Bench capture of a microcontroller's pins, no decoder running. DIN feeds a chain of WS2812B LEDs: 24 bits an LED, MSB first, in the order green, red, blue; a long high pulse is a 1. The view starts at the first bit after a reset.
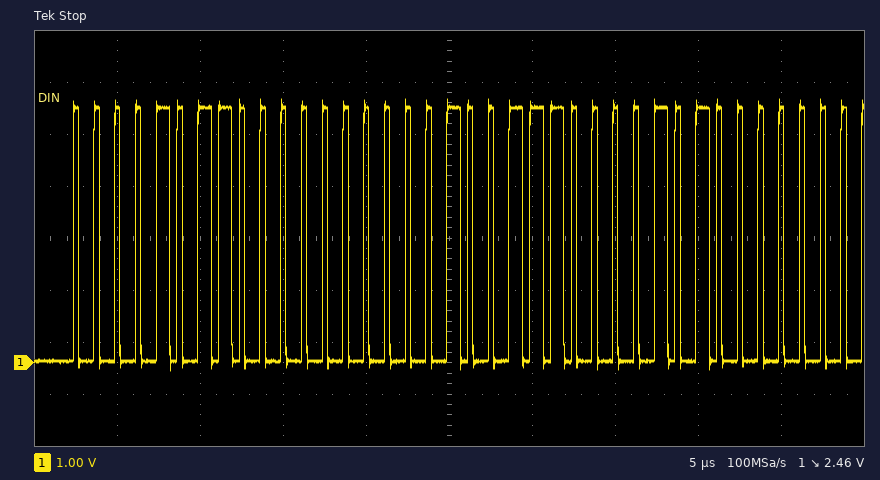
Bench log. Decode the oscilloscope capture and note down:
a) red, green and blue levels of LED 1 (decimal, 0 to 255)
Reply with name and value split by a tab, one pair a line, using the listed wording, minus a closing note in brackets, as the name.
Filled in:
red, green and blue levels of LED 1	0, 11, 39
